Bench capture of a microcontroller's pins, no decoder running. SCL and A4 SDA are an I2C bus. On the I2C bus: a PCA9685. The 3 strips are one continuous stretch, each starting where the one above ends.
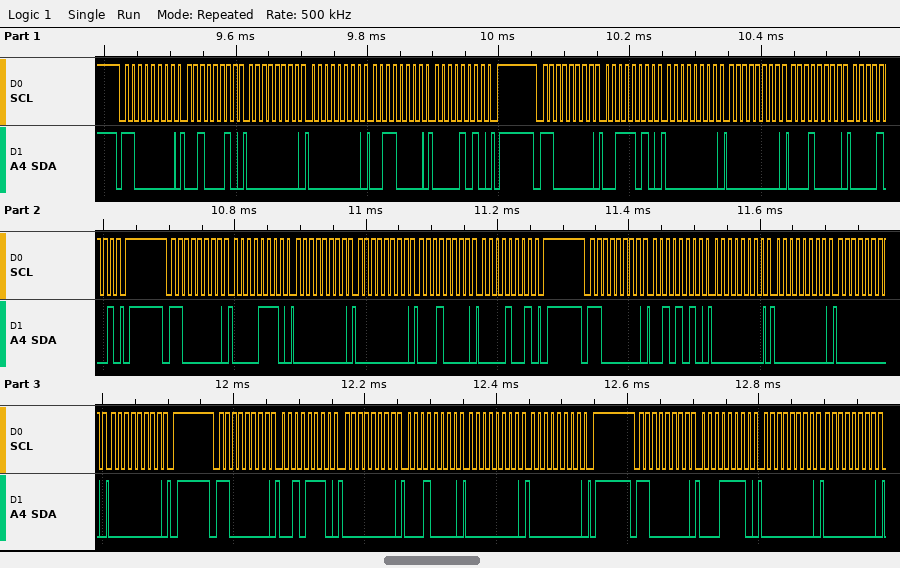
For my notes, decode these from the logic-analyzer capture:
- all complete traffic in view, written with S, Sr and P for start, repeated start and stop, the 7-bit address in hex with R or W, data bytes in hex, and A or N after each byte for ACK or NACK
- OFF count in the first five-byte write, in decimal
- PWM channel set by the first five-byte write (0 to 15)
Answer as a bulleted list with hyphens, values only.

- S 60W A 22 A 00 A 00 A 30 A 0A A P S 60W A 3A A 00 A 00 A 10 A 09 A P S 60W A 0E A 00 A 00 A 10 A 09 A P S 60W A 2A A 00 A 00 A 00 A 00 A P S 60W A 2E A 00 A 10 A 00 A 00 A P S 60W A 1E A 00 A 00 A
- 2608
- 7
